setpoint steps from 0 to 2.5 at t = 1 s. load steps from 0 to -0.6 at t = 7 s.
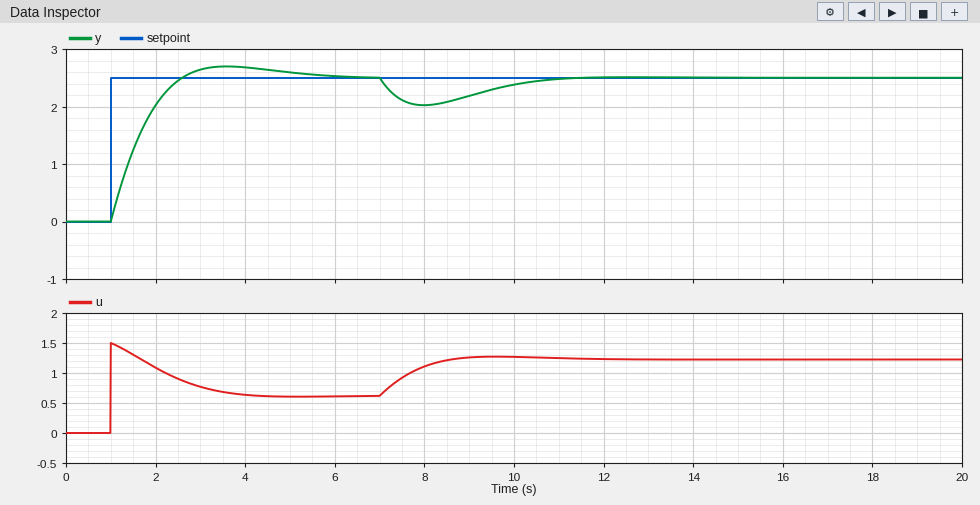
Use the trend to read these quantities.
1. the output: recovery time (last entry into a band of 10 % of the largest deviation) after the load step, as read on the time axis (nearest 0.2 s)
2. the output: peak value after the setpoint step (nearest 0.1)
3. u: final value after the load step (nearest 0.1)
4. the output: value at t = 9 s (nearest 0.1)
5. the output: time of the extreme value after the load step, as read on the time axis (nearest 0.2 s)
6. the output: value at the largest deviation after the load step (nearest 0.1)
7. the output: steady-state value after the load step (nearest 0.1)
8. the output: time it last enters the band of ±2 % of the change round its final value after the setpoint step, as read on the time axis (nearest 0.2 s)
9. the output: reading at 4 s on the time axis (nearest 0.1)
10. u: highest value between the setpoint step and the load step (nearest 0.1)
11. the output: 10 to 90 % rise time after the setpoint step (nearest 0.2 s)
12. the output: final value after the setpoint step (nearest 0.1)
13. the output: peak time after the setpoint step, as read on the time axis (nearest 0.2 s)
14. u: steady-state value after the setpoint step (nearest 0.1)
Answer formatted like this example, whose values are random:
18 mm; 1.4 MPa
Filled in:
10.6 s; 2.7; 1.2; 2.2; 8.0 s; 2.0; 2.5; 5.6 s; 2.7; 1.5; 1.2 s; 2.5; 3.6 s; 0.6
